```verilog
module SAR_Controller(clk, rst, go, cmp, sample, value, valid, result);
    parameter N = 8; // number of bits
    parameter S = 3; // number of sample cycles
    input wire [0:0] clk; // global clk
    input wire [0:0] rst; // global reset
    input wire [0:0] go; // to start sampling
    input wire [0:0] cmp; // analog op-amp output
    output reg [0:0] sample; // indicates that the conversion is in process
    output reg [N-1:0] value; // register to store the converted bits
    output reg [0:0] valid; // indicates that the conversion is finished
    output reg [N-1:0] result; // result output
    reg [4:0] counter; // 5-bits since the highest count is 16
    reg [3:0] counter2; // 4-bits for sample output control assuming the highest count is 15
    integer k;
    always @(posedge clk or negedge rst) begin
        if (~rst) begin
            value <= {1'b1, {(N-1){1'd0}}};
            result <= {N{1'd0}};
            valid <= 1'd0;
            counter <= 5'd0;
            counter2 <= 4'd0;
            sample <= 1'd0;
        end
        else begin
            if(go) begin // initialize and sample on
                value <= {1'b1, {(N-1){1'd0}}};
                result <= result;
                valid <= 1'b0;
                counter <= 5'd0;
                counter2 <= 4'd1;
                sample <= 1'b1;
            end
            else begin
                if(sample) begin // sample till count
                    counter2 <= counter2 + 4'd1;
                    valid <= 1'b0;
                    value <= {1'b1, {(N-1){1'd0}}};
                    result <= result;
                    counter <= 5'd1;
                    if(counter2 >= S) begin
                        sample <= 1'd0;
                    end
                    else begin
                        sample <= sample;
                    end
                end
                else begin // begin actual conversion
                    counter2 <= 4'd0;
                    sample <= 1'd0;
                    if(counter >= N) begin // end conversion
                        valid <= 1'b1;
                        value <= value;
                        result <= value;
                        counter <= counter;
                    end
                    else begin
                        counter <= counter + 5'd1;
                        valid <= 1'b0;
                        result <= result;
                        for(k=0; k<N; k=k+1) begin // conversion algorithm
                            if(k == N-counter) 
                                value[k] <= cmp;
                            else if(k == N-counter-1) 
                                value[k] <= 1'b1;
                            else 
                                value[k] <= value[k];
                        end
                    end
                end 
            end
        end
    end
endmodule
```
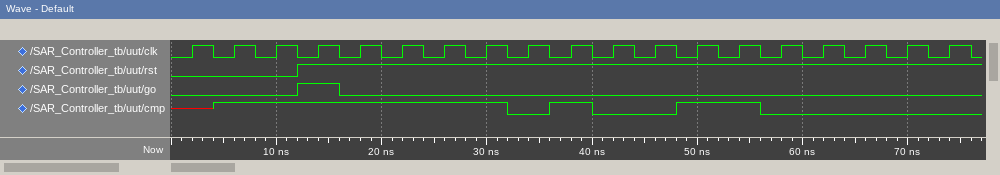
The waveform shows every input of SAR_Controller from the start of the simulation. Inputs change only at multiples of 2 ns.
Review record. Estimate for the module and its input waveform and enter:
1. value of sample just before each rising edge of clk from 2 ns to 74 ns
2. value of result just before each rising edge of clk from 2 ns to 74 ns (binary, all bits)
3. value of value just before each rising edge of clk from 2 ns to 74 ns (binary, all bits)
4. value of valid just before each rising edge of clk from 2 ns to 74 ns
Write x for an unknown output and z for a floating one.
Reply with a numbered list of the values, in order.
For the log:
1. 0 0 0 0 1 1 1 0 0 0 0 0 0 0 0 0 0 0 0
2. 00000000, 00000000, 00000000, 00000000, 00000000, 00000000, 00000000, 00000000, 00000000, 00000000, 00000000, 00000000, 00000000, 00000000, 00000000, 10100111, 10100111, 10100111, 10100111
3. 10000000, 10000000, 10000000, 10000000, 10000000, 10000000, 10000000, 10000000, 11000000, 10100000, 10110000, 10101000, 10100100, 10100110, 10100111, 10100111, 10100111, 10100111, 10100111
4. 0 0 0 0 0 0 0 0 0 0 0 0 0 0 0 1 1 1 1
